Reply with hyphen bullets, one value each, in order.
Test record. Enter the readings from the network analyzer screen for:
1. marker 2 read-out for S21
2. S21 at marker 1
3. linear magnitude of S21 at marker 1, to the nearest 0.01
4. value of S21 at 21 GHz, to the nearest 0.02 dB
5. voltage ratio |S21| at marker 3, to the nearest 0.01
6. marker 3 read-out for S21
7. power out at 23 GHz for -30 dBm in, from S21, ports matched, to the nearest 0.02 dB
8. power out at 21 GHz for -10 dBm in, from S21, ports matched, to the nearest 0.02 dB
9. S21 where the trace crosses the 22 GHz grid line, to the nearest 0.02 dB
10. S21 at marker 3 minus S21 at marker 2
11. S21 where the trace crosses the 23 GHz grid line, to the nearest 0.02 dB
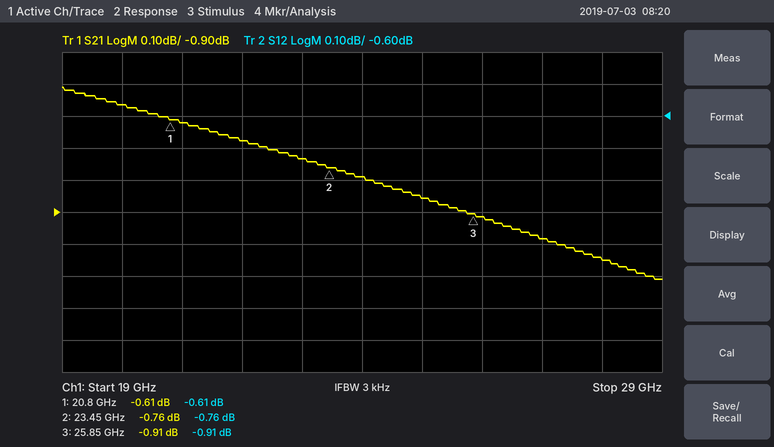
- -0.76 dB
- -0.61 dB
- 0.93
- -0.62 dB
- 0.90
- -0.91 dB
- -30.74 dBm
- -10.62 dBm
- -0.68 dB
- -0.15 dB
- -0.74 dB
